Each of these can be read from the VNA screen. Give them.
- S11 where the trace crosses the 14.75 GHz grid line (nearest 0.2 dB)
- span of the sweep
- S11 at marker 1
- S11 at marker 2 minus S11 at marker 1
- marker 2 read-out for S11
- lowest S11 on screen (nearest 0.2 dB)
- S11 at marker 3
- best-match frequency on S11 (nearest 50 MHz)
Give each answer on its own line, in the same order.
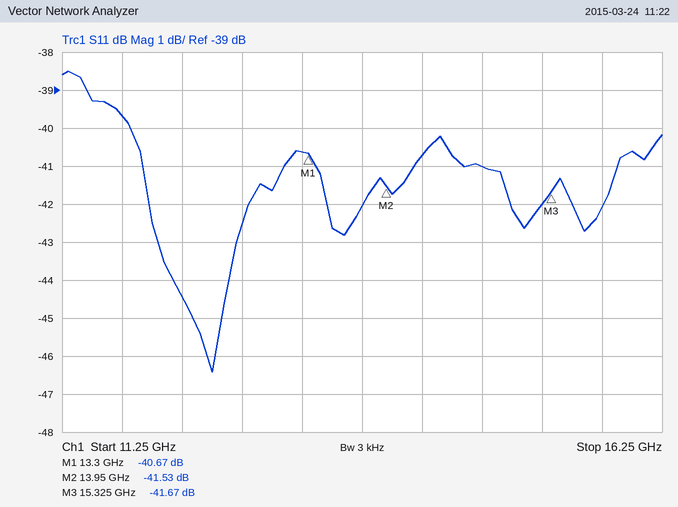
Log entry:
-41.0 dB
5 GHz
-40.67 dB
-0.86 dB
-41.53 dB
-46.4 dB
-41.67 dB
12.50 GHz
